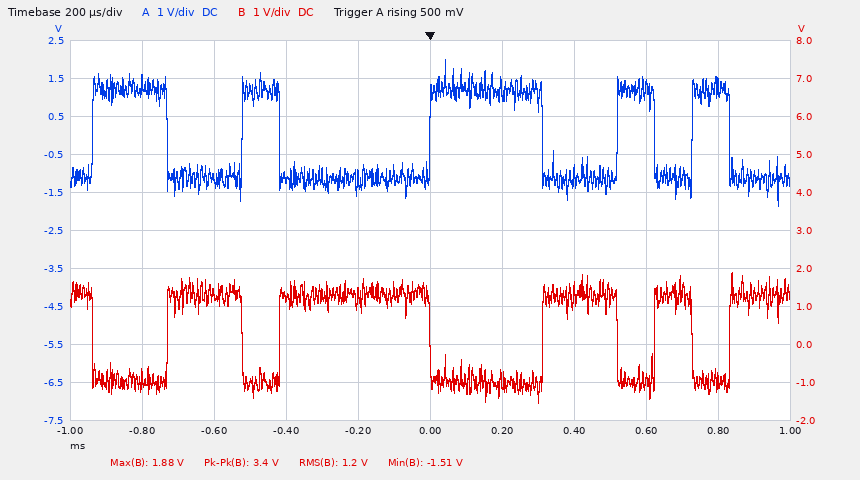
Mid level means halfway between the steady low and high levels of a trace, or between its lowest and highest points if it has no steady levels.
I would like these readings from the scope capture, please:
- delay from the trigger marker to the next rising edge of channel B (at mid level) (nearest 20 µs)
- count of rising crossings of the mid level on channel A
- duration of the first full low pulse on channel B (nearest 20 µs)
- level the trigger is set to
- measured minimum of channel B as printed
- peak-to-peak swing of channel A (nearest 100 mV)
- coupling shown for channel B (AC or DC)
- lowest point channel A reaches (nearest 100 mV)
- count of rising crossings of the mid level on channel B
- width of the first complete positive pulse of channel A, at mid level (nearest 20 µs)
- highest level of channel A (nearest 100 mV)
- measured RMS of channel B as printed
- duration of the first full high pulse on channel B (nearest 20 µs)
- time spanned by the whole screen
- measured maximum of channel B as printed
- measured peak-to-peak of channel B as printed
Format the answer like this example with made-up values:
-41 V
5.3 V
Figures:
320 µs
5
200 µs
500 mV
-1.51 V
3.8 V
DC
-1.8 V
5
200 µs
2.0 V
1.2 V
200 µs
2 ms
1.88 V
3.4 V
